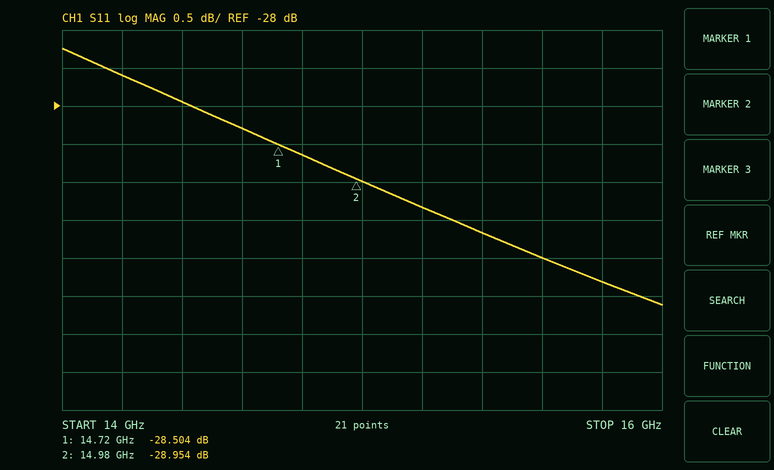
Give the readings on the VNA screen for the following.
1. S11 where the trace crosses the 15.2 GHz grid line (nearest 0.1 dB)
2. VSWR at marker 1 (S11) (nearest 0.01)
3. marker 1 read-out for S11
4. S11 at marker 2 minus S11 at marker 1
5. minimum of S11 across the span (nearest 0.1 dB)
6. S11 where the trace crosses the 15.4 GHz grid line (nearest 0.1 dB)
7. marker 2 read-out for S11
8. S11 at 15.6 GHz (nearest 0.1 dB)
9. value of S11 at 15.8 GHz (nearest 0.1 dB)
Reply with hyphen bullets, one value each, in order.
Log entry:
- -29.3 dB
- 1.08
- -28.504 dB
- -0.450 dB
- -30.6 dB
- -29.7 dB
- -28.954 dB
- -30.0 dB
- -30.3 dB
